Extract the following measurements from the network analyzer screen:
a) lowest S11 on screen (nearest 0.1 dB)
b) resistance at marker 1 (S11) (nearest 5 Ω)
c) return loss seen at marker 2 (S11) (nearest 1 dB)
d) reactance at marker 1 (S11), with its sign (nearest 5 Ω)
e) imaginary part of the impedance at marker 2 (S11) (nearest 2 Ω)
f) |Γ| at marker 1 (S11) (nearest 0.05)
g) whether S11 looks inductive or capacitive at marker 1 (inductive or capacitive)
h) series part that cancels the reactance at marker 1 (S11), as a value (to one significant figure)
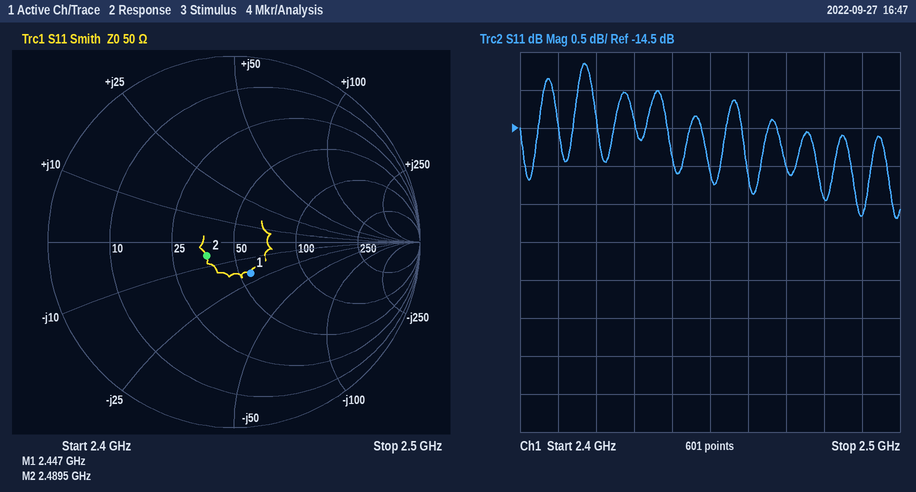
-15.7 dB
55 Ω
16 dB
-20 Ω
-6 Ω
0.20
capacitive
1 nH
